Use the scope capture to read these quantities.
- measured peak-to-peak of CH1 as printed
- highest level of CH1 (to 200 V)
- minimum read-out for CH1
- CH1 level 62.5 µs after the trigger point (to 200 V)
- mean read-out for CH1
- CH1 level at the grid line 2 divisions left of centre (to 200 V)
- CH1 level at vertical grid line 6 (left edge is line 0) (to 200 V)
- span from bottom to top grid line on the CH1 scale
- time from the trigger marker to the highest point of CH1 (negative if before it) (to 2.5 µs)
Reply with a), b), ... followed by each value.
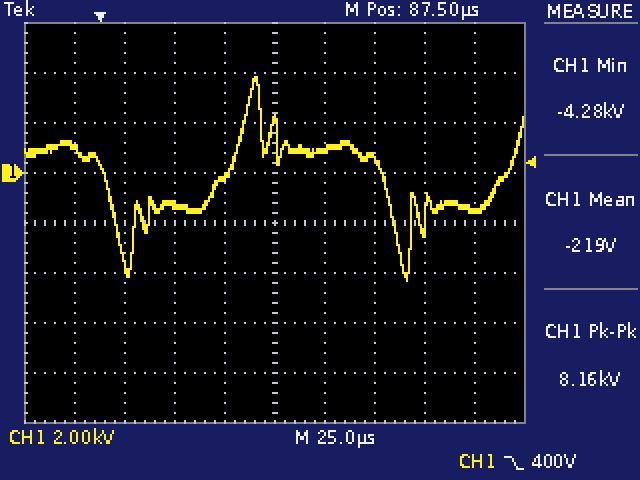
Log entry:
a) 8.16 kV
b) 3.8 kV
c) -4.28 kV
d) -200 V
e) -219 V
f) -1.2 kV
g) 1.0 kV
h) 16 kV
i) +77.5 µs
